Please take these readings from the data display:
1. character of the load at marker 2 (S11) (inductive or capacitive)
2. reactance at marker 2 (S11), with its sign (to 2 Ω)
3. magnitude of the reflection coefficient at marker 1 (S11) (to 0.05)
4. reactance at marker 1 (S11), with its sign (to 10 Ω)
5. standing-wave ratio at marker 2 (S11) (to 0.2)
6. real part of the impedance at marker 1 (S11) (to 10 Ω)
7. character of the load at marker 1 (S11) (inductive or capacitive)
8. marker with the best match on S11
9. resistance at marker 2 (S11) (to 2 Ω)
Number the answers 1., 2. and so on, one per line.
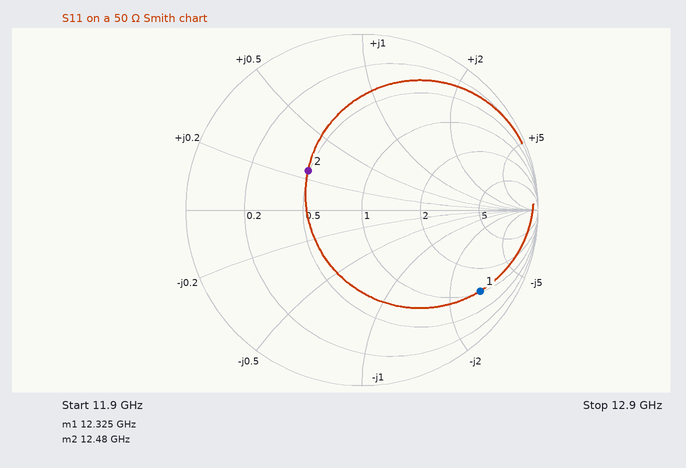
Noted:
1. inductive
2. +12 Ω
3. 0.80
4. -140 Ω
5. 2.2
6. 50 Ω
7. capacitive
8. marker 2
9. 24 Ω
